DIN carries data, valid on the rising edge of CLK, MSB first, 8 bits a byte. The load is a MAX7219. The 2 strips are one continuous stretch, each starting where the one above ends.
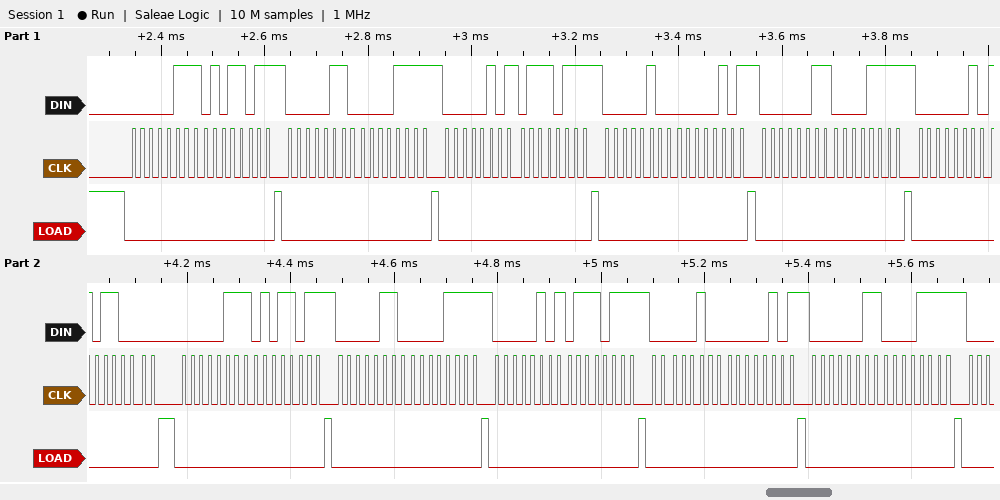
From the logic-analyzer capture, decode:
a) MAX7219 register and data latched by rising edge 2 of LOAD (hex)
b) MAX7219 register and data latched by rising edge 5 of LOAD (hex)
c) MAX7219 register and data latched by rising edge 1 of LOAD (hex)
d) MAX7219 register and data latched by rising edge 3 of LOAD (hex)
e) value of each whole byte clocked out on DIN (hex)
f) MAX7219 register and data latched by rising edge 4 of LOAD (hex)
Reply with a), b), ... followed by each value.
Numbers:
a) register 0x6, data 0x0F
b) register 0x3, data 0x0F
c) register 0x7, data 0x5B
d) register 0x5, data 0x77
e) 07 5B 06 0F 05 77 04 05 03 0F 02 B0 07 5B 06 0F 05 77 04 05 03 0F
f) register 0x4, data 0x05
